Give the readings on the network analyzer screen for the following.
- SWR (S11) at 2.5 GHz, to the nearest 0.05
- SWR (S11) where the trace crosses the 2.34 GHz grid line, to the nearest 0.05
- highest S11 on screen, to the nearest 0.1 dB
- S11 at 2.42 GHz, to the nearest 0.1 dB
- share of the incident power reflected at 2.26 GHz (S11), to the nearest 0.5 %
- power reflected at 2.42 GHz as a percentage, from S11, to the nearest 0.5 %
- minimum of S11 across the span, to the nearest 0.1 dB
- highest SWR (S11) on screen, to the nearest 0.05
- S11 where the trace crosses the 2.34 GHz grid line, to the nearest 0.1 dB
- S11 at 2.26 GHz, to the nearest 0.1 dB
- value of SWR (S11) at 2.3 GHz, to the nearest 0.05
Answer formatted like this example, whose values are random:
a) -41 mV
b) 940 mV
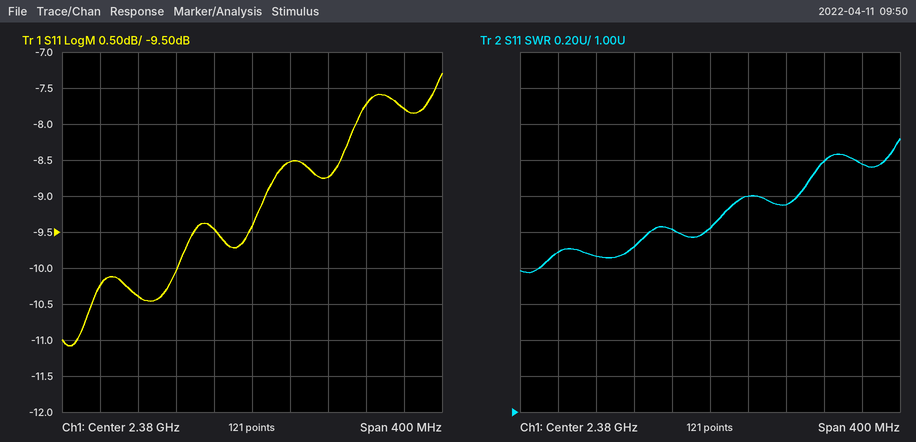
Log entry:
a) 2.40
b) 2.00
c) -7.3 dB
d) -8.5 dB
e) 9.0 %
f) 14.0 %
g) -11.1 dB
h) 2.50
i) -9.5 dB
j) -10.4 dB
k) 1.90
